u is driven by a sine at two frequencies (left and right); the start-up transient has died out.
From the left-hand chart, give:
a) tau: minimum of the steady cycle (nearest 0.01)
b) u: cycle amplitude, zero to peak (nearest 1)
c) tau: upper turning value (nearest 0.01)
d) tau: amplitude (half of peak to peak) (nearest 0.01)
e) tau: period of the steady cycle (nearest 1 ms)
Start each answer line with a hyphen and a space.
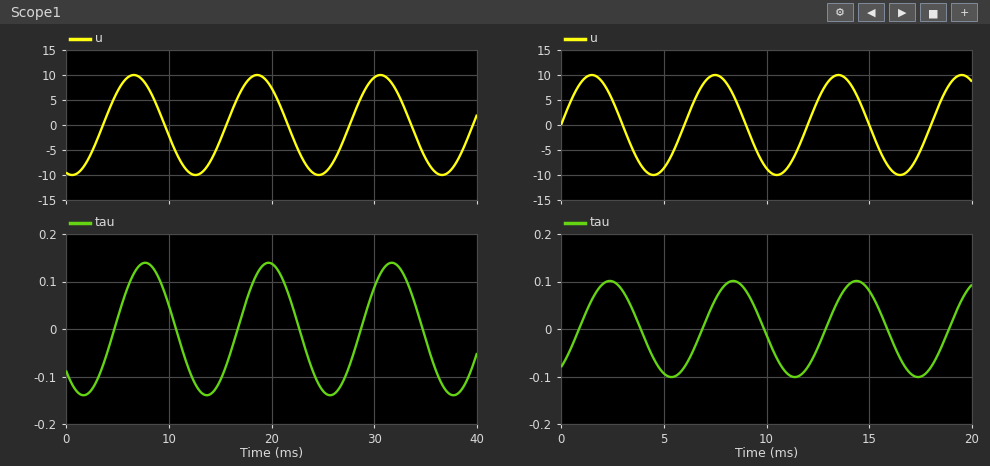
- -0.14
- 10
- 0.14
- 0.14
- 12 ms
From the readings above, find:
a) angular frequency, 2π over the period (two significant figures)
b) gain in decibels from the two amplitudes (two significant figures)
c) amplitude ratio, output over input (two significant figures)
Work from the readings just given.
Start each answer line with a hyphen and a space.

- 0.52 rad/ms
- -37 dB
- 0.014
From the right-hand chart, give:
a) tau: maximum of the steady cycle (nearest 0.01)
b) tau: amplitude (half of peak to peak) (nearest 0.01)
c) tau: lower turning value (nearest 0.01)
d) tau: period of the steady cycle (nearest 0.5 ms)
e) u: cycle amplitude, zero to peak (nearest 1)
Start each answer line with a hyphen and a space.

- 0.10
- 0.10
- -0.10
- 6.0 ms
- 10
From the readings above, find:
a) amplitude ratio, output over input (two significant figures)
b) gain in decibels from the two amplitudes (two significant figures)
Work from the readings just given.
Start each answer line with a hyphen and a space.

- 0.010
- -40 dB
